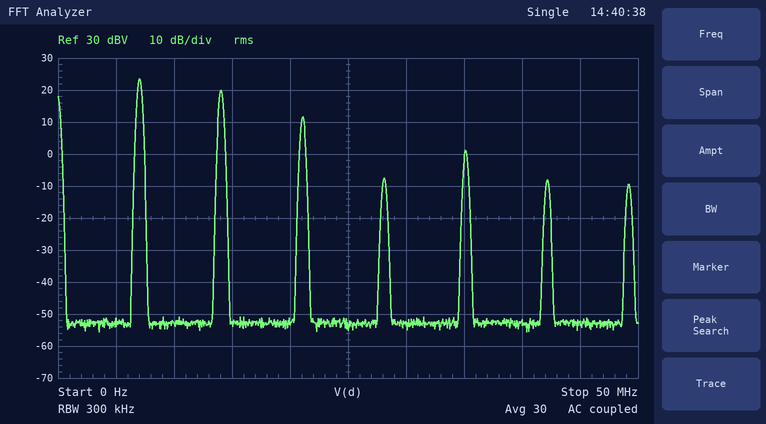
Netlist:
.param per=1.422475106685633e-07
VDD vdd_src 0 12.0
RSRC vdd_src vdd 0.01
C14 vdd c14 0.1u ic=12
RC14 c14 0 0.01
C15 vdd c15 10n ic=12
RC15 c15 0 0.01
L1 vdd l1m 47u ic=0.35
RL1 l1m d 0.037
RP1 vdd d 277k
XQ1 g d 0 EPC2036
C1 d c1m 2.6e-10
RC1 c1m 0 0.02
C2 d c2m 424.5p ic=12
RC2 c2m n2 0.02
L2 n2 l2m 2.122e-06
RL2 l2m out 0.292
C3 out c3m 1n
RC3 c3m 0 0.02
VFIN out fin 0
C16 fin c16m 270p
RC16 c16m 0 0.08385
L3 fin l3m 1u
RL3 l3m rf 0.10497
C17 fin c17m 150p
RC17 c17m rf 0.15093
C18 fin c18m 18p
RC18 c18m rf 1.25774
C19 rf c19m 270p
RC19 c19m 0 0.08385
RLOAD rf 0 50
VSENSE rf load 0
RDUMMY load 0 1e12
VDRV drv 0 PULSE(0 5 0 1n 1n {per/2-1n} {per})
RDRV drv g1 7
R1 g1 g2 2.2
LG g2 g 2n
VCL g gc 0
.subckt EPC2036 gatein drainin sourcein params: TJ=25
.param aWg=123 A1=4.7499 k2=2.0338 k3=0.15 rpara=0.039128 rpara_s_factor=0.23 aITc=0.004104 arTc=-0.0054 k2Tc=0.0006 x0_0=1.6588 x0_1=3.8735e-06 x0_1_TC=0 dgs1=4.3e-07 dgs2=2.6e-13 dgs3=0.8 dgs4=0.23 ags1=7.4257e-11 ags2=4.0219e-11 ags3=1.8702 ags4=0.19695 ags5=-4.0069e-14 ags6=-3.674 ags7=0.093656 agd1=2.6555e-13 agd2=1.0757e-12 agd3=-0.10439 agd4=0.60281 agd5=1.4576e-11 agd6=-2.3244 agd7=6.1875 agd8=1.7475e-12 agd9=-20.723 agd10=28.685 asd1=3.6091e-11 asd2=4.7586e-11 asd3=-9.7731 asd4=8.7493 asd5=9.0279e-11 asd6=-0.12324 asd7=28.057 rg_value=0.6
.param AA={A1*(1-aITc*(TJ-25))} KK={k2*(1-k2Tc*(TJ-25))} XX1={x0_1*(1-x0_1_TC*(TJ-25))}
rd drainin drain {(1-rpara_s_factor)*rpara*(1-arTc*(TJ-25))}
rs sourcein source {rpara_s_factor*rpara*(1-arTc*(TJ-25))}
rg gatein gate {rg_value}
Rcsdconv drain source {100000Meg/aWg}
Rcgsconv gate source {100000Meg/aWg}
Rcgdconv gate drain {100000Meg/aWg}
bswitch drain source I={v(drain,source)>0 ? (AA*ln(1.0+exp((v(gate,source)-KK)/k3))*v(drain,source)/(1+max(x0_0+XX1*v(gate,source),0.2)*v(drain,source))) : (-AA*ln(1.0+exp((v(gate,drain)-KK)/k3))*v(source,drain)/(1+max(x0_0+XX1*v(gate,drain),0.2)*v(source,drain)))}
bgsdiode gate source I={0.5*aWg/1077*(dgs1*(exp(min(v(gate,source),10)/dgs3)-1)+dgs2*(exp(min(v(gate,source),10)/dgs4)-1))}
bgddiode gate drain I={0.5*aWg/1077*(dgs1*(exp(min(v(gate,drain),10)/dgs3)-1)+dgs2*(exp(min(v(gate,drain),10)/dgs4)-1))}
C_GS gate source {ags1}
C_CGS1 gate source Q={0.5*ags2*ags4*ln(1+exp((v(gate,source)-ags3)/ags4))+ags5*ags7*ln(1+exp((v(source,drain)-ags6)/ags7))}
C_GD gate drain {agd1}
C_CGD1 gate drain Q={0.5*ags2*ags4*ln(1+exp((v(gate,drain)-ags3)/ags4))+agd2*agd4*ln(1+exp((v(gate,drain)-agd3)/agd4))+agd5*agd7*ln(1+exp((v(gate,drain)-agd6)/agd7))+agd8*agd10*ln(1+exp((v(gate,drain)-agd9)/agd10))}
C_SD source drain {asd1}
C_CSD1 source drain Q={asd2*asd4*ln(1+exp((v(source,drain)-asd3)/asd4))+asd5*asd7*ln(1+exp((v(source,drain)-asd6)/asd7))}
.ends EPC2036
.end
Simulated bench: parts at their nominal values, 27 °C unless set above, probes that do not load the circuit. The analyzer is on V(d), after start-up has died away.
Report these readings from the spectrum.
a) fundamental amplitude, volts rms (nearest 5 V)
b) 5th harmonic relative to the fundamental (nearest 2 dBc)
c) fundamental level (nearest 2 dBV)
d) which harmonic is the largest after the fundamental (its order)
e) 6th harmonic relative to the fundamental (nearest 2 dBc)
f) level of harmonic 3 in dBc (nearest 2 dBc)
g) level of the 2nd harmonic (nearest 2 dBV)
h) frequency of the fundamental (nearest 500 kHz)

15 V
-22 dBc
24 dBV
2
-32 dBc
-12 dBc
20 dBV
7.0 MHz
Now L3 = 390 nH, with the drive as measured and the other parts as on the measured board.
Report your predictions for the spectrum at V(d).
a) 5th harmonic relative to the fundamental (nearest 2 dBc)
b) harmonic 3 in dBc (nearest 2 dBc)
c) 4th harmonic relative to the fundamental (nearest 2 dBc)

-26 dBc
-18 dBc
-24 dBc
